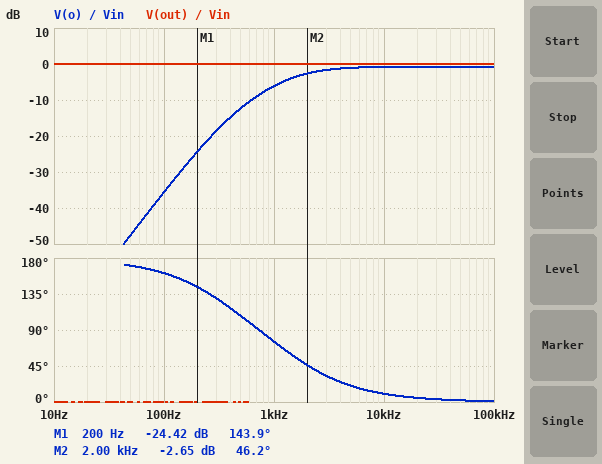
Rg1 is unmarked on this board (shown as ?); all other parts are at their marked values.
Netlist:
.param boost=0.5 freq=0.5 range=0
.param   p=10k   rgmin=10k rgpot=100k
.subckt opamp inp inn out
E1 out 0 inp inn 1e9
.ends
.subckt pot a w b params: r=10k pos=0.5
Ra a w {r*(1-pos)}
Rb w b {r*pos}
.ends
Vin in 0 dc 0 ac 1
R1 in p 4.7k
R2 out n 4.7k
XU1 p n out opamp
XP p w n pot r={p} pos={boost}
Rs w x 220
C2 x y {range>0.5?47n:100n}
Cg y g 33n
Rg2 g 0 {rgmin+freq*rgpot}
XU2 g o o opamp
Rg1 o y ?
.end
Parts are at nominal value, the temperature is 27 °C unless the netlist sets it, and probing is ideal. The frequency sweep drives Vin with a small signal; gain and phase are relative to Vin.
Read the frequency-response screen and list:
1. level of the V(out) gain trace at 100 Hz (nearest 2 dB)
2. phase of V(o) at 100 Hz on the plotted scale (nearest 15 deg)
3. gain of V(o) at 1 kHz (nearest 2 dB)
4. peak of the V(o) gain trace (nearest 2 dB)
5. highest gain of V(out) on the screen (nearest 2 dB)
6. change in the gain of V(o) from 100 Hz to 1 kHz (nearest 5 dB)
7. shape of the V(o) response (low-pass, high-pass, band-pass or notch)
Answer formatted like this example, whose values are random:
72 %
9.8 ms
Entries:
0 dB
165 deg
-6 dB
0 dB
0 dB
30 dB
high-pass
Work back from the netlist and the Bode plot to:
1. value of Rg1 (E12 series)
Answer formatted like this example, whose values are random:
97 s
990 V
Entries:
220 Ω
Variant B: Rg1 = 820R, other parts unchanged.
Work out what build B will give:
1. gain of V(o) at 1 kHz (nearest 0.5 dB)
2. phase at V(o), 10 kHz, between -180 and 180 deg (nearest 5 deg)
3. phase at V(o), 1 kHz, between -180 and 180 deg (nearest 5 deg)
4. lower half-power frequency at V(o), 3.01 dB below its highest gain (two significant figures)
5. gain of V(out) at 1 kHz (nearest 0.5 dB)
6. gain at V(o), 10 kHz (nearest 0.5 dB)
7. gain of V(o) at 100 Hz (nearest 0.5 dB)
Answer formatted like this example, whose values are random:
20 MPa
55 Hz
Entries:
-1.0 dB
5 deg
35 deg
390 Hz
0 dB
-0.5 dB
-24.0 dB
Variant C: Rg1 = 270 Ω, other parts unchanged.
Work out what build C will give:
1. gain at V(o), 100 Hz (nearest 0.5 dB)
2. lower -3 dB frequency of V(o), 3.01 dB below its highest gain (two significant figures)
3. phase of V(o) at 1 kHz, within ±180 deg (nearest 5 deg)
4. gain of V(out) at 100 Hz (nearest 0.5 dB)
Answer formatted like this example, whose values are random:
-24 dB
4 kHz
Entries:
-34.0 dB
1.2 kHz
70 deg
0 dB
